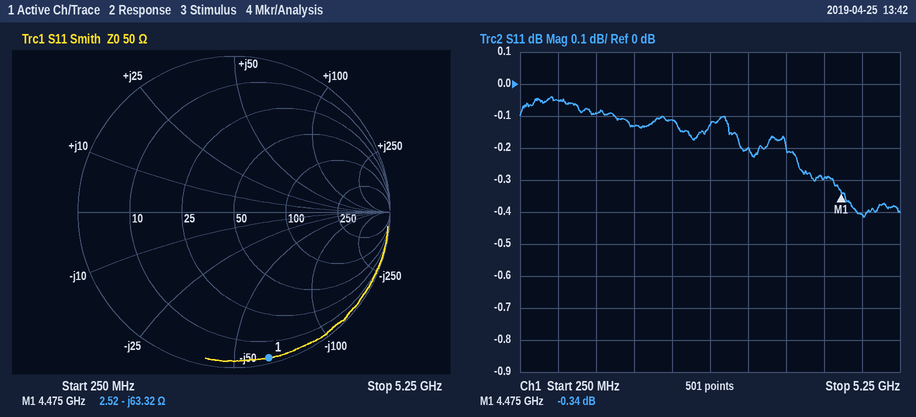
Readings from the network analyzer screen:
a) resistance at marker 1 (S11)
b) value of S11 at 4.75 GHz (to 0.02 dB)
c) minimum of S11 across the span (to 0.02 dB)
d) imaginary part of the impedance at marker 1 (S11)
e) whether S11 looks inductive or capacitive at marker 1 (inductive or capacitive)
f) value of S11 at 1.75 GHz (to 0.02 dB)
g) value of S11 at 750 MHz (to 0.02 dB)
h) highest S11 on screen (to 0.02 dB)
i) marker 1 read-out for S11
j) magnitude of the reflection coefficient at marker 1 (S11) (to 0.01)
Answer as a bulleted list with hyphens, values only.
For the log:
- 2.52 Ω
- -0.40 dB
- -0.42 dB
- -63.32 Ω
- capacitive
- -0.14 dB
- -0.06 dB
- -0.04 dB
- -0.34 dB
- 0.96
